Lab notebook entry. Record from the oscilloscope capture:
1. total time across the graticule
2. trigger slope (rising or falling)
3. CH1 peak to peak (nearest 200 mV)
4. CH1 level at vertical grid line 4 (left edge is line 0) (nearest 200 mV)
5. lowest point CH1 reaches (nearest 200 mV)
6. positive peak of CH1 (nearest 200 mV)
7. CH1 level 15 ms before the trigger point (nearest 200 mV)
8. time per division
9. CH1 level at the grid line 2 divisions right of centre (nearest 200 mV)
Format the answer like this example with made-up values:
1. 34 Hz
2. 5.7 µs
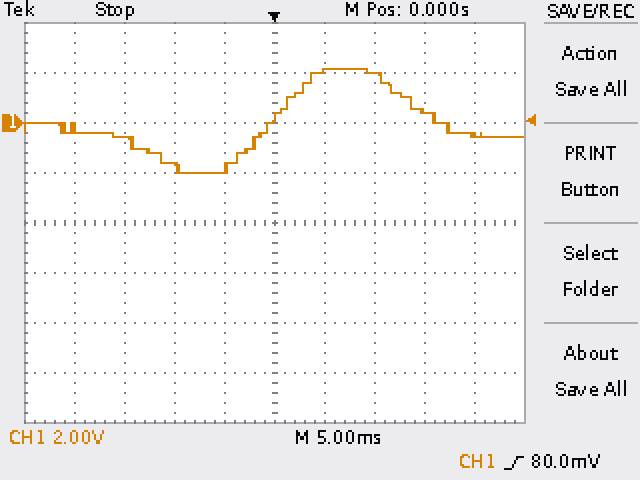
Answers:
1. 50 ms
2. rising
3. 4.2 V
4. -1.8 V
5. -2.0 V
6. 2.2 V
7. -600 mV
8. 5 ms
9. 2.0 V
